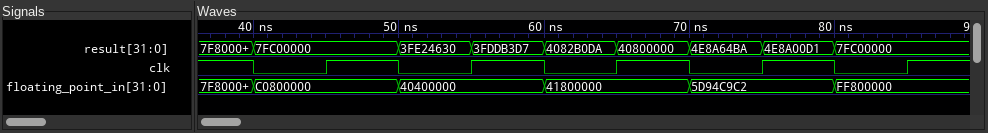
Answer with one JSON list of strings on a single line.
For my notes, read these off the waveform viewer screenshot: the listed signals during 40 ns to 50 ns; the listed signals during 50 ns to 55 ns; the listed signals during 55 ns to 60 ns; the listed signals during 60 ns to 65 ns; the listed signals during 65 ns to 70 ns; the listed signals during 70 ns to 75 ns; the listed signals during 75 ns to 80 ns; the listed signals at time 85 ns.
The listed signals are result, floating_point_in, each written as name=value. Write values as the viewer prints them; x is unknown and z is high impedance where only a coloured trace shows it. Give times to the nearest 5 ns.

["result=7FC00000, floating_point_in=C0800000", "result=3FE24630, floating_point_in=40400000", "result=3FDDB3D7, floating_point_in=40400000", "result=4082B0DA, floating_point_in=41800000", "result=40800000, floating_point_in=41800000", "result=4E8A64BA, floating_point_in=5D94C9C2", "result=4E8A00D1, floating_point_in=5D94C9C2", "result=7FC00000, floating_point_in=FF800000"]
